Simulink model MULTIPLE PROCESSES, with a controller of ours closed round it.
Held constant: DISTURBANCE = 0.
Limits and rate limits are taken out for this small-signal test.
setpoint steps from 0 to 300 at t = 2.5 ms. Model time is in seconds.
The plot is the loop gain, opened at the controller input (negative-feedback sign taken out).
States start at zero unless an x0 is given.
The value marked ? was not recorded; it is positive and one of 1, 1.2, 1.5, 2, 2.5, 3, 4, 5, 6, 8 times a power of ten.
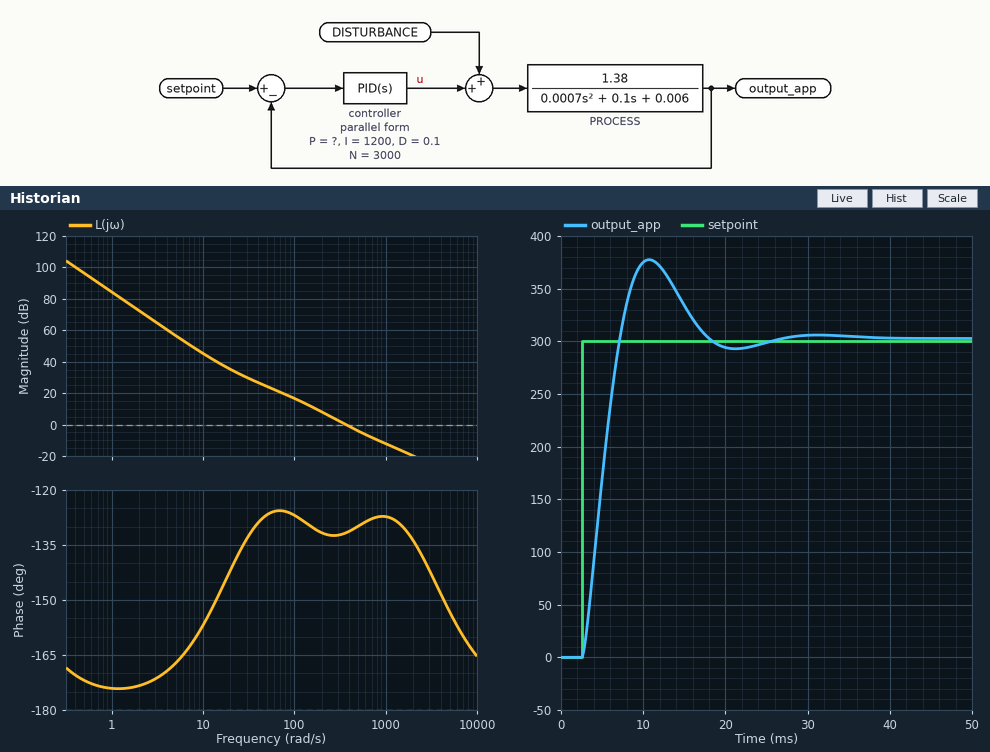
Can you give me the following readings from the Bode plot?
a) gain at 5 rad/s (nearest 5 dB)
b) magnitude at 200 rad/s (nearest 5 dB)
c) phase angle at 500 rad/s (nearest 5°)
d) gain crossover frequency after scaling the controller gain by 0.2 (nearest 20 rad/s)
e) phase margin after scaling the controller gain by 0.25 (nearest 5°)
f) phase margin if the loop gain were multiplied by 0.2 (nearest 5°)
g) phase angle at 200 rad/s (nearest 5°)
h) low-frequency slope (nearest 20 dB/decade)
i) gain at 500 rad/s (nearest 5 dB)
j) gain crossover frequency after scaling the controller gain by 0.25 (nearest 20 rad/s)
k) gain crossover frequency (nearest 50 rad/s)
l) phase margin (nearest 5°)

55 dB
10 dB
-130°
120 rad/s
50°
50°
-130°
-40 dB/decade
-5 dB
140 rad/s
350 rad/s
50°
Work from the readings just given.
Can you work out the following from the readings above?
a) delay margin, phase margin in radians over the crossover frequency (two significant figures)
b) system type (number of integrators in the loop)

0.0025 s
2
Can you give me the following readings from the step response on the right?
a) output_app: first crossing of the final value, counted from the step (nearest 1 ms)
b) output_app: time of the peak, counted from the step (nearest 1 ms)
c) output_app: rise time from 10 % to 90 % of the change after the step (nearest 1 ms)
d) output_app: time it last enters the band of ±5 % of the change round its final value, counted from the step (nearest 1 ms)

5 ms
8 ms
3 ms
14 ms
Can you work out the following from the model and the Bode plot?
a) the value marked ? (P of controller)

60
